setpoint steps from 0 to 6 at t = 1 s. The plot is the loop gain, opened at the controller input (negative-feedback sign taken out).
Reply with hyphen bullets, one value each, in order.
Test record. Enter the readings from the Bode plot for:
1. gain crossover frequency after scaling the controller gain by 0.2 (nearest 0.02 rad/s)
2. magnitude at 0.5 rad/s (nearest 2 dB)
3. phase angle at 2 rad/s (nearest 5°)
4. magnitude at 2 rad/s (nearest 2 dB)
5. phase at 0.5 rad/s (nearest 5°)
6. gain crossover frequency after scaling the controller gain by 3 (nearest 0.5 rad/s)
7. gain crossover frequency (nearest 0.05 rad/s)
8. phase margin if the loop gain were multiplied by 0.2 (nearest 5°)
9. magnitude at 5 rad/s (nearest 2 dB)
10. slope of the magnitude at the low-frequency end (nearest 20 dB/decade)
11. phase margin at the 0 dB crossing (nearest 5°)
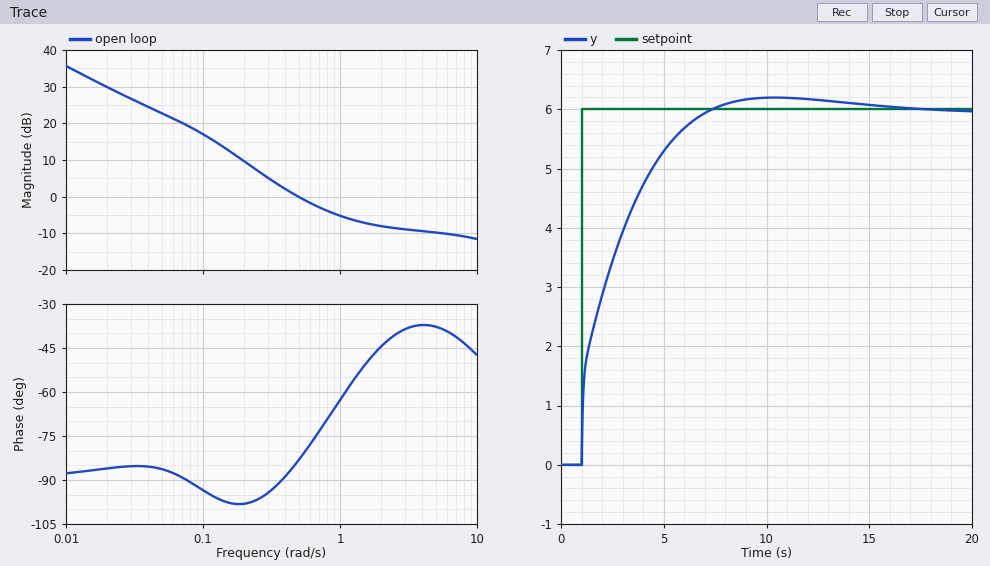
- 0.14 rad/s
- 0 dB
- -45°
- -8 dB
- -85°
- 4.5 rad/s
- 0.50 rad/s
- 85°
- -10 dB
- -20 dB/decade
- 95°
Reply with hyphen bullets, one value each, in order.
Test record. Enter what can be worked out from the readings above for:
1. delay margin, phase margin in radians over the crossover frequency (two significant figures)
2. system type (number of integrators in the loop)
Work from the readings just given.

- 3.3 s
- 1
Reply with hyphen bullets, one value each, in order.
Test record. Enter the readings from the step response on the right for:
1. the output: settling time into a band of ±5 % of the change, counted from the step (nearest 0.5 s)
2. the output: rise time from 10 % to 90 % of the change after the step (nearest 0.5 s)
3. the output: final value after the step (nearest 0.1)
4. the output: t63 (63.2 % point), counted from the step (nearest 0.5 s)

- 5.0 s
- 4.0 s
- 6.0
- 2.0 s
